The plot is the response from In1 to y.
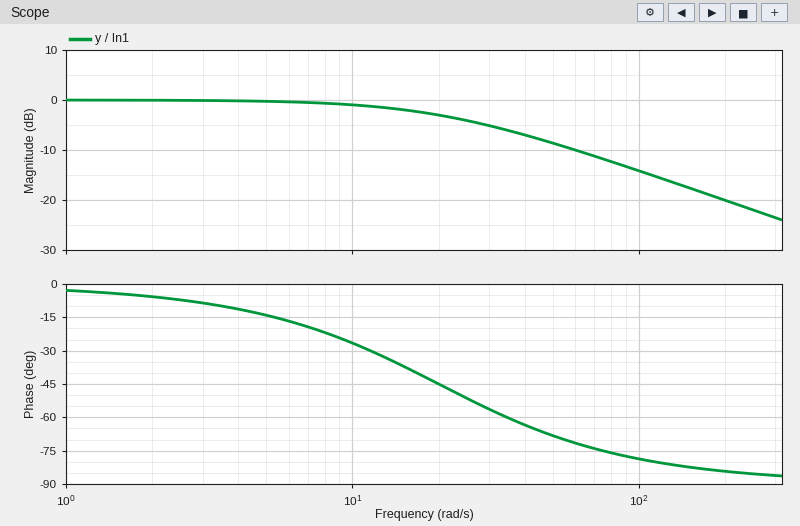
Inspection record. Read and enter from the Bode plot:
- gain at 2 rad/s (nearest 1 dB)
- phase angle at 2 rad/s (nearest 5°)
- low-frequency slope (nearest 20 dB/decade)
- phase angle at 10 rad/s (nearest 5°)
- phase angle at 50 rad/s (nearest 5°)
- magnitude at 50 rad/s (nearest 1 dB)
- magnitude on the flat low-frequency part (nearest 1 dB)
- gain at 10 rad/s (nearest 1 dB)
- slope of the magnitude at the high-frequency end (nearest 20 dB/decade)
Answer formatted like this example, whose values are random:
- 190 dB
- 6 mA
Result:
- 0 dB
- -5°
- 0 dB/decade
- -25°
- -70°
- -9 dB
- 0 dB
- -1 dB
- -20 dB/decade
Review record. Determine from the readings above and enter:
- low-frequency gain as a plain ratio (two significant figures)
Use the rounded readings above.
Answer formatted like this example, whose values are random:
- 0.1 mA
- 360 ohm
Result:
- 1.0
